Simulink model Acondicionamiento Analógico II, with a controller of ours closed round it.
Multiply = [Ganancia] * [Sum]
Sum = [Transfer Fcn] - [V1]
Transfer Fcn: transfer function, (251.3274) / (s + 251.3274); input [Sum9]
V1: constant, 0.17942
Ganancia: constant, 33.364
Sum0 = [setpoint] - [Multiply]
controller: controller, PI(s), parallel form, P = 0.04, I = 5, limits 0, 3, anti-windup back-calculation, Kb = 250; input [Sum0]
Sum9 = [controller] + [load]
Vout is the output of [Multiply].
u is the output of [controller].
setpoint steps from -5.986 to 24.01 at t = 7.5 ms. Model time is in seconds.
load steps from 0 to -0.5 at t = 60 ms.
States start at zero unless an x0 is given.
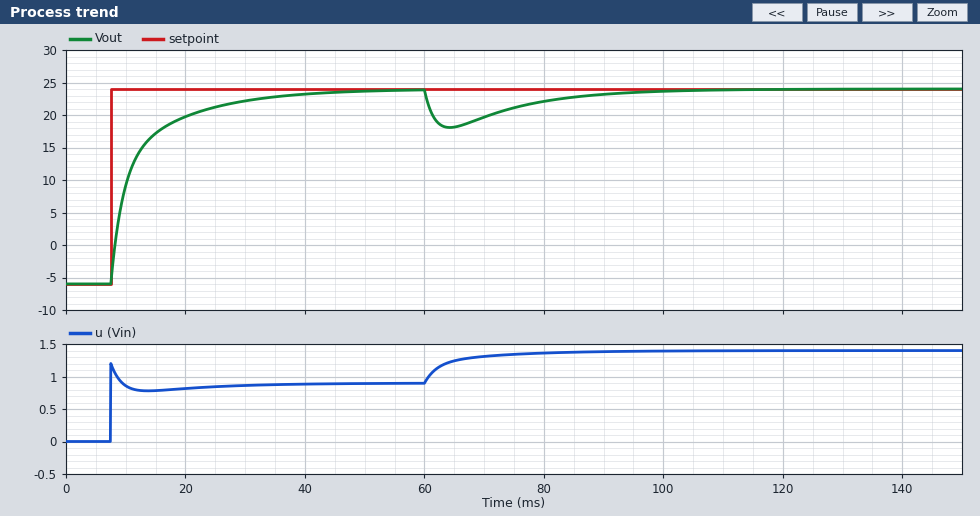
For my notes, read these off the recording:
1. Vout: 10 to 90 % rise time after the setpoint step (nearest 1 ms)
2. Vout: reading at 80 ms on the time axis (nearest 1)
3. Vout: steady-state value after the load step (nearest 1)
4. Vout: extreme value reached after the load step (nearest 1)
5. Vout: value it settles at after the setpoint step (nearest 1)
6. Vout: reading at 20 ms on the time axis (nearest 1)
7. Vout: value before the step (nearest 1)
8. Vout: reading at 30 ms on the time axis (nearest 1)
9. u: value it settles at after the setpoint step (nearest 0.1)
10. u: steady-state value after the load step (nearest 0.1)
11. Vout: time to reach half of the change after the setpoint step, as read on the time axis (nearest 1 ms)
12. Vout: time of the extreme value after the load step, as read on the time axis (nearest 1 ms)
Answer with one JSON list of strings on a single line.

["16 ms", "22", "24", "18", "24", "20", "-6", "22", "0.9", "1.4", "10 ms", "64 ms"]
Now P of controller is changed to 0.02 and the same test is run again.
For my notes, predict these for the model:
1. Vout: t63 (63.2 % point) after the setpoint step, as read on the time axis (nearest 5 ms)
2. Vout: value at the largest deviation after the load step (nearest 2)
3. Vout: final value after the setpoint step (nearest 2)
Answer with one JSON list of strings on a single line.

["15 ms", "16", "24"]
